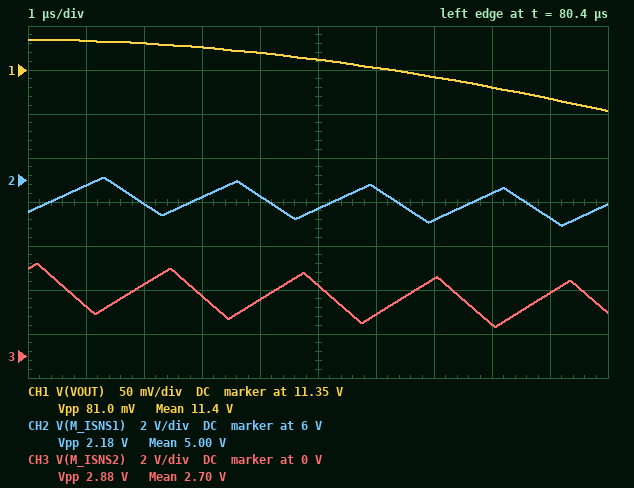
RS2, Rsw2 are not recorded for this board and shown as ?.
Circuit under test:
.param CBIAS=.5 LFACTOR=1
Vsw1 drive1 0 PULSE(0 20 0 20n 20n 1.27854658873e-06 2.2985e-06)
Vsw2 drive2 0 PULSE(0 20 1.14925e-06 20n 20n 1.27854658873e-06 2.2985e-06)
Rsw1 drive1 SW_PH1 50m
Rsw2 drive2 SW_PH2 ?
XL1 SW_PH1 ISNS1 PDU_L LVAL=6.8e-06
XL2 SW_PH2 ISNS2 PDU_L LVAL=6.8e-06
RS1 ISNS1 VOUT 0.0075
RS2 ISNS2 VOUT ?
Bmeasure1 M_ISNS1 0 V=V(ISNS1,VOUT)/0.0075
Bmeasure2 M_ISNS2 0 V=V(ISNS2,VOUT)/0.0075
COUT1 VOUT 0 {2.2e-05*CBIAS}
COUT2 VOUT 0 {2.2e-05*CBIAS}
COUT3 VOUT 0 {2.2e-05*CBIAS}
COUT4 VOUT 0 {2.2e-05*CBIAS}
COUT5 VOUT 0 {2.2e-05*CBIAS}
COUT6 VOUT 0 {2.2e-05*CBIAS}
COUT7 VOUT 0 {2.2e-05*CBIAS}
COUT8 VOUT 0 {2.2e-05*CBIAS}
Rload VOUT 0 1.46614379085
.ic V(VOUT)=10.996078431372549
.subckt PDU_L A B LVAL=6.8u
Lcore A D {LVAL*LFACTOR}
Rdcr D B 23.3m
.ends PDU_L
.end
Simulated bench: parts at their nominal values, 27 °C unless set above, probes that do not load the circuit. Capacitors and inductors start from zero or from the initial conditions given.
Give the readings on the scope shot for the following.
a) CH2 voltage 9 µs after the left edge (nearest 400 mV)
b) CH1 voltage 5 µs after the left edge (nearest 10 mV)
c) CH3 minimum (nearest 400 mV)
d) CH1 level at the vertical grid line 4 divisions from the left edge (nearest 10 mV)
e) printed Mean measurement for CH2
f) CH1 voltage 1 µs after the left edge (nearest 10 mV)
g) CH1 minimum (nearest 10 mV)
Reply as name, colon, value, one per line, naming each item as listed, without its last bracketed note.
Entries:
CH2 voltage 9 µs after the left edge: 4.4 V
CH1 voltage 5 µs after the left edge: 11.36 V
CH3 minimum: 1.2 V
CH1 level at the vertical grid line 4 divisions from the left edge: 11.37 V
printed Mean measurement for CH2: 5.00 V
CH1 voltage 1 µs after the left edge: 11.38 V
CH1 minimum: 11.30 V
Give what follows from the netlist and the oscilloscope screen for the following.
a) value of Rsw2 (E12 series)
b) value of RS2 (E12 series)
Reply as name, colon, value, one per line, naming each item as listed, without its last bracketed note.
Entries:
value of Rsw2: 0.15 Ω
value of RS2: 0.01 Ω
